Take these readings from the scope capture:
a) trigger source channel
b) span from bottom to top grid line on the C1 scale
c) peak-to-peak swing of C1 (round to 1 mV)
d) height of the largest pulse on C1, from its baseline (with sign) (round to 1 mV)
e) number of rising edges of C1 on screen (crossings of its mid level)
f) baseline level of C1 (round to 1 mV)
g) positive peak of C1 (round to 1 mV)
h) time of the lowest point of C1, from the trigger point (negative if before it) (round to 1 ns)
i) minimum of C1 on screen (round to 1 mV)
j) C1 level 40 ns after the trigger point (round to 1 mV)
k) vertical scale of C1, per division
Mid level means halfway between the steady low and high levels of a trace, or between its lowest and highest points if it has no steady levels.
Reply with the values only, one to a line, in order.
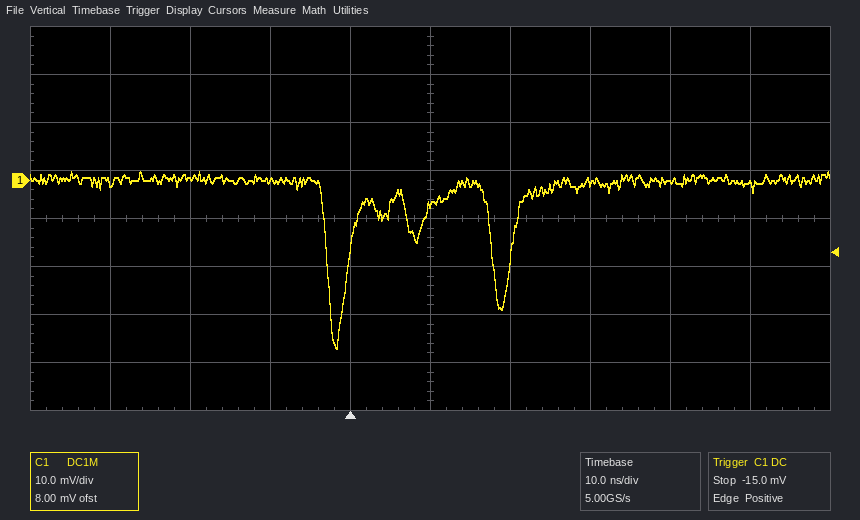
C1
80 mV
37 mV
-35 mV
2
0 mV
2 mV
-2 ns
-35 mV
0 mV
10 mV
